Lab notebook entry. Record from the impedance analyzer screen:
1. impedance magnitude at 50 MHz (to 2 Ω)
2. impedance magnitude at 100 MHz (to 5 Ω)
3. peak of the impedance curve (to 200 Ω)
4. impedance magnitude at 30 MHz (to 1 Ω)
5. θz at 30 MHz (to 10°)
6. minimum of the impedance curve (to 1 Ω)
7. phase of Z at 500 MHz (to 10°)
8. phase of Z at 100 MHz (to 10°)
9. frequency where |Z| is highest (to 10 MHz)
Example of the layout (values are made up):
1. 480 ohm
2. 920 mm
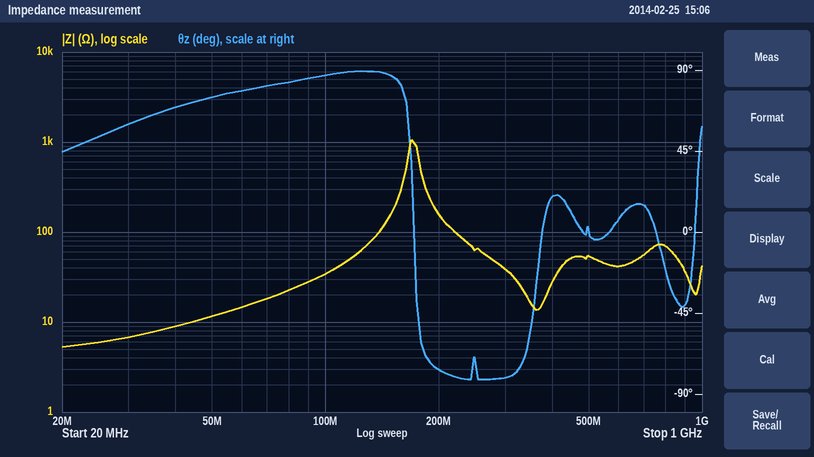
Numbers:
1. 12 Ω
2. 35 Ω
3. 1.0 kΩ
4. 7 Ω
5. 60°
6. 5 Ω
7. 0°
8. 90°
9. 170 MHz
